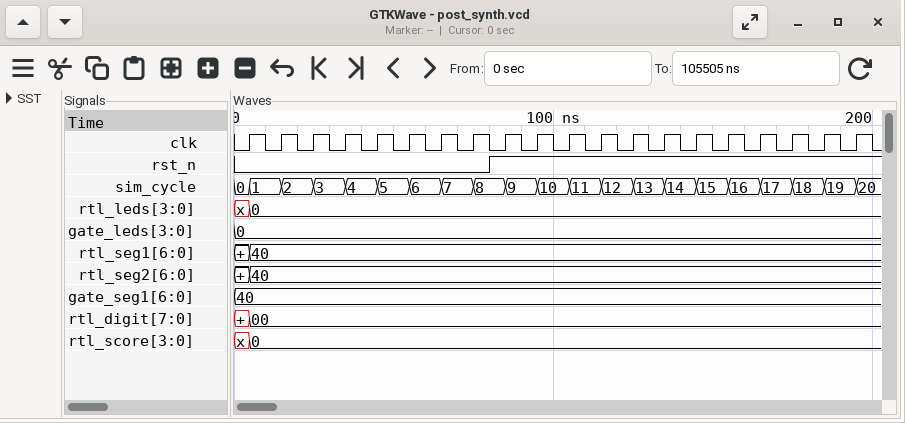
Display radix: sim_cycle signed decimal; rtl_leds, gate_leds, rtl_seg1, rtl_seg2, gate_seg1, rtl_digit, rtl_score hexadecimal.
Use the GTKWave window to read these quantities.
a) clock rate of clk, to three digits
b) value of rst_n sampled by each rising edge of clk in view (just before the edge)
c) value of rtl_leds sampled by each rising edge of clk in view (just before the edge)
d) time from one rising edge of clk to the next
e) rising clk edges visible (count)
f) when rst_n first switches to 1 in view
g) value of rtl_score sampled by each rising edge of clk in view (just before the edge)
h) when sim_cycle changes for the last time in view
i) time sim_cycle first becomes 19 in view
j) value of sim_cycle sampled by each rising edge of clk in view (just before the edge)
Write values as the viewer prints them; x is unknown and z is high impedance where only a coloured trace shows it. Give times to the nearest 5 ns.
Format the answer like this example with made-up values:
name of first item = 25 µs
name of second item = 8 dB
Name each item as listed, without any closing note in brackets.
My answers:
clock rate of clk, to three digits = 100 MHz
value of rst_n sampled by each rising edge of clk in view = 0 0 0 0 0 0 0 0 1 1 1 1 1 1 1 1 1 1 1 1
value of rtl_leds sampled by each rising edge of clk in view = x, 0, 0, 0, 0, 0, 0, 0, 0, 0, 0, 0, 0, 0, 0, 0, 0, 0, 0, 0
time from one rising edge of clk to the next = 10 ns
rising clk edges visible = 20
when rst_n first switches to 1 in view = 80 ns
value of rtl_score sampled by each rising edge of clk in view = x, 0, 0, 0, 0, 0, 0, 0, 0, 0, 0, 0, 0, 0, 0, 0, 0, 0, 0, 0
when sim_cycle changes for the last time in view = 195 ns
time sim_cycle first becomes 19 in view = 185 ns
value of sim_cycle sampled by each rising edge of clk in view = 0, 1, 2, 3, 4, 5, 6, 7, 8, 9, 10, 11, 12, 13, 14, 15, 16, 17, 18, 19
